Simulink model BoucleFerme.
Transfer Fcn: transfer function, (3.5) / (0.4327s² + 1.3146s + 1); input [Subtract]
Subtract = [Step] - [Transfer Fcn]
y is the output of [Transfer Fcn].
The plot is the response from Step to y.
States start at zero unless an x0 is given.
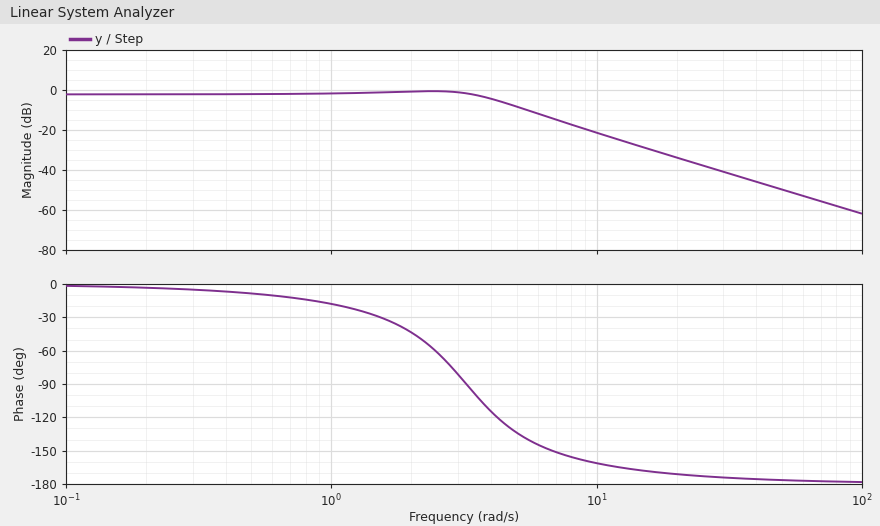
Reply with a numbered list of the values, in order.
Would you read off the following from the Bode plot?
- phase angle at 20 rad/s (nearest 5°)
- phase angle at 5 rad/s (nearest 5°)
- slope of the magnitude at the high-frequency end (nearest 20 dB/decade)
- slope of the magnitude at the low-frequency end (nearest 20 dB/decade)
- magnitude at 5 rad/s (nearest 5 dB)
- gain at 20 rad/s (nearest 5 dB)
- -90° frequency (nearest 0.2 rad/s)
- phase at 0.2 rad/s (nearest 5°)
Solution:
1. -170°
2. -135°
3. -40 dB/decade
4. 0 dB/decade
5. -10 dB
6. -35 dB
7. 3.2 rad/s
8. -5°
